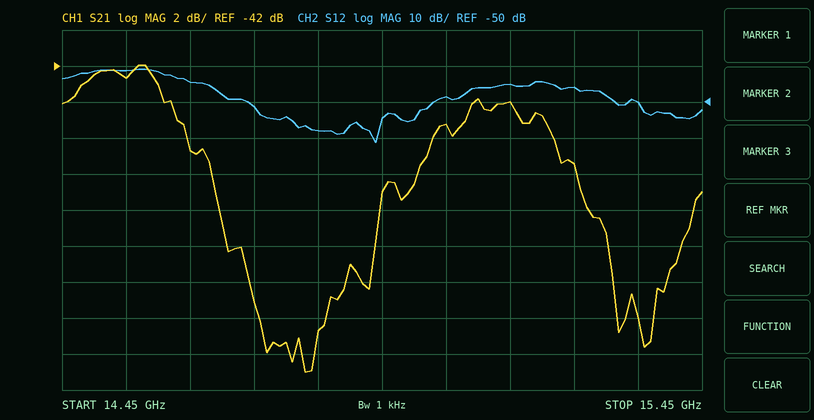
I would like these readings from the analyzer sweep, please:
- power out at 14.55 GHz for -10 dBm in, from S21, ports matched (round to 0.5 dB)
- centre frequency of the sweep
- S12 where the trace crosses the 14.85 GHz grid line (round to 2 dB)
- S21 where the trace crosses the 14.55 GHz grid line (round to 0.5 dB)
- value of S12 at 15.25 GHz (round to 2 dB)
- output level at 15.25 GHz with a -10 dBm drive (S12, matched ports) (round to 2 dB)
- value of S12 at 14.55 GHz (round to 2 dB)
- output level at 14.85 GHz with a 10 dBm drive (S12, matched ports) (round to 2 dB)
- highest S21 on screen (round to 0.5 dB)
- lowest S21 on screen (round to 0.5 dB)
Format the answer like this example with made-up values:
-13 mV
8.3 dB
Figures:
-52.5 dBm
14.95 GHz
-58 dB
-42.5 dB
-46 dB
-56 dBm
-42 dB
-48 dBm
-42.0 dB
-59.0 dB
